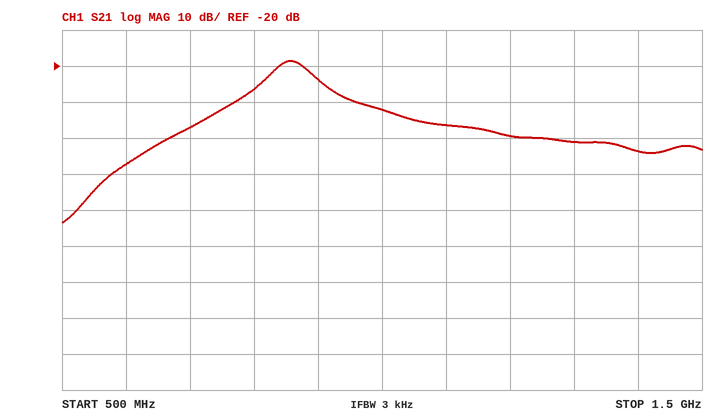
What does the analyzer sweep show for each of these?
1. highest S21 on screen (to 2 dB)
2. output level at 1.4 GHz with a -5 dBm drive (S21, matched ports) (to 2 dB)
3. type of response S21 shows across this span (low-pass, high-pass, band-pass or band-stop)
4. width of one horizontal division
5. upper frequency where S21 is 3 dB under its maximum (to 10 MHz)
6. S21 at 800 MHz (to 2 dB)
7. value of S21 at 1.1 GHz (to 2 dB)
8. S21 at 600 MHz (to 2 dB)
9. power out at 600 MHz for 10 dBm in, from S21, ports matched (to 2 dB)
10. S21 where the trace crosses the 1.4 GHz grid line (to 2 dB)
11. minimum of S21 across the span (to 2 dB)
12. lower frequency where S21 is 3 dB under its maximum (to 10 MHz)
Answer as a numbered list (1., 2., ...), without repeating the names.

1. -18 dB
2. -48 dBm
3. band-pass
4. 100 MHz
5. 890 MHz
6. -26 dB
7. -36 dB
8. -48 dB
9. -38 dBm
10. -44 dB
11. -64 dB
12. 830 MHz
